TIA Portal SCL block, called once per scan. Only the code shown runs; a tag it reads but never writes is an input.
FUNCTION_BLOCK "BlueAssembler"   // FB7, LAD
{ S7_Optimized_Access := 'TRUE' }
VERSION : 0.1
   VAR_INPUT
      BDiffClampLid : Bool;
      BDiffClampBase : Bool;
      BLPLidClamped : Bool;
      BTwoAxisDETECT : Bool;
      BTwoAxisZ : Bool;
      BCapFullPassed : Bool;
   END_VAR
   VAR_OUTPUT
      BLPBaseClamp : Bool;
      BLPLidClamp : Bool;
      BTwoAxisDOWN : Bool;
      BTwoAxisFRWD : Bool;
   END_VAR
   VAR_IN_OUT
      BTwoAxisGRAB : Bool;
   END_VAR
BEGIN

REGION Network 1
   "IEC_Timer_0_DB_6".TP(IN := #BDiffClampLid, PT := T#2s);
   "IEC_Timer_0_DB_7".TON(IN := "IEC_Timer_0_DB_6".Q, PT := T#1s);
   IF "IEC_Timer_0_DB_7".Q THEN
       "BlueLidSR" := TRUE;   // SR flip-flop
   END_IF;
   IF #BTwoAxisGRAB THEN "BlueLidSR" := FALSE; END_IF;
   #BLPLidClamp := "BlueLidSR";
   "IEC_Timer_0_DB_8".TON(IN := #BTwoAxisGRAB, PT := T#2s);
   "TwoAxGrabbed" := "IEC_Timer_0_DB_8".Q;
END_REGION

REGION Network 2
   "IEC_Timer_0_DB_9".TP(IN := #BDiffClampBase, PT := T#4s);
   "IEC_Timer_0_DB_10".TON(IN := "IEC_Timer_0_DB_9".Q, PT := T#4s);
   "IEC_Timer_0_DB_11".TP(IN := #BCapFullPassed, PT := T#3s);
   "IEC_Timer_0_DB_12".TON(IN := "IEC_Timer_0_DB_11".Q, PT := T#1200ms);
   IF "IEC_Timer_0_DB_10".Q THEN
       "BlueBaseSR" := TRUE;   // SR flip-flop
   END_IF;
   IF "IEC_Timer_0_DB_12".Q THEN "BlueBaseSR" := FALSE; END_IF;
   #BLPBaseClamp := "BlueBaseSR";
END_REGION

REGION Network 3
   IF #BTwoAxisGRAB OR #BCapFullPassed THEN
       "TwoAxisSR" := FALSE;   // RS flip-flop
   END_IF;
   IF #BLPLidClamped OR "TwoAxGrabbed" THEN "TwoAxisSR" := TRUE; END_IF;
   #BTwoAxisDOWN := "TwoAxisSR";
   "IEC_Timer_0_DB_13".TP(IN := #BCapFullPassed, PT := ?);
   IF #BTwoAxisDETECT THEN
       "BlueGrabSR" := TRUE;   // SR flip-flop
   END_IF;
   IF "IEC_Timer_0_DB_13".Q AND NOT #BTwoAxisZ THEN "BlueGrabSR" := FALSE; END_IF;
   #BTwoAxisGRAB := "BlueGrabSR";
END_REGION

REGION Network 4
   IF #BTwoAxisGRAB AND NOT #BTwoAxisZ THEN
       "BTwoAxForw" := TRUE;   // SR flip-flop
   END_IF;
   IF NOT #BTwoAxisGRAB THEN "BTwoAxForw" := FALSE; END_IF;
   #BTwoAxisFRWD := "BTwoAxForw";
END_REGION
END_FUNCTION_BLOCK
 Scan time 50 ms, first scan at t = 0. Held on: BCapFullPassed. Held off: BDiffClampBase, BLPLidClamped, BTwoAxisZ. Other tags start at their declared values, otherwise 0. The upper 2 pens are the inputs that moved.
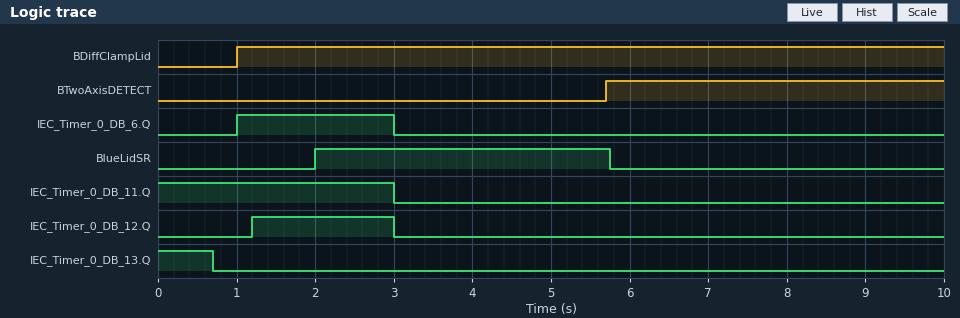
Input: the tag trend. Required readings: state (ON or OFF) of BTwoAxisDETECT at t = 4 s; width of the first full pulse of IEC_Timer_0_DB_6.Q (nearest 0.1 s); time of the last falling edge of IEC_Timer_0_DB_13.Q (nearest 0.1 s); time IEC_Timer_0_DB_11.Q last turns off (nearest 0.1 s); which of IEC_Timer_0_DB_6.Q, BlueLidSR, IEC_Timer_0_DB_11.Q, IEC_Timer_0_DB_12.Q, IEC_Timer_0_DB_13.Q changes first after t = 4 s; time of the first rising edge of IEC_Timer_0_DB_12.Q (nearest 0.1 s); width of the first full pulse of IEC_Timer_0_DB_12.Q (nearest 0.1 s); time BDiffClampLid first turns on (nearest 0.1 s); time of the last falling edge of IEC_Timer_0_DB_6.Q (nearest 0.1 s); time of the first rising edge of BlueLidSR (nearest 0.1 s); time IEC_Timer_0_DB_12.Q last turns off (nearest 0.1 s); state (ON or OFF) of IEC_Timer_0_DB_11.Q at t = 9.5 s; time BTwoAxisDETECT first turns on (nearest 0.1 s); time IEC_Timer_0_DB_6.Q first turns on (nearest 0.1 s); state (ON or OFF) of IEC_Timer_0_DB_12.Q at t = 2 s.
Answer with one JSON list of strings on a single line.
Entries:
["OFF", "2.0 s", "0.7 s", "3.0 s", "BlueLidSR", "1.2 s", "1.8 s", "1.0 s", "3.0 s", "2.0 s", "3.0 s", "OFF", "5.7 s", "1.0 s", "ON"]
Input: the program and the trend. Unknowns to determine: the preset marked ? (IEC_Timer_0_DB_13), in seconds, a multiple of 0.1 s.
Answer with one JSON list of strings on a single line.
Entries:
["0.7 s"]
